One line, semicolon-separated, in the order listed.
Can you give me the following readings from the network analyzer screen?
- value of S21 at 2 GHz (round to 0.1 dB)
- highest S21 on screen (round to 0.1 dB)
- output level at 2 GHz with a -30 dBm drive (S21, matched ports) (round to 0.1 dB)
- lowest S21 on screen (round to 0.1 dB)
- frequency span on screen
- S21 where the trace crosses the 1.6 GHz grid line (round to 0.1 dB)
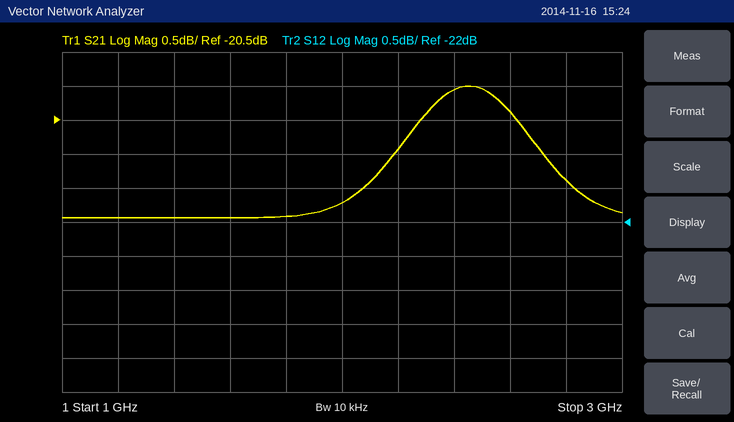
-21.7 dB; -20.0 dB; -51.7 dBm; -21.9 dB; 2 GHz; -21.9 dB
